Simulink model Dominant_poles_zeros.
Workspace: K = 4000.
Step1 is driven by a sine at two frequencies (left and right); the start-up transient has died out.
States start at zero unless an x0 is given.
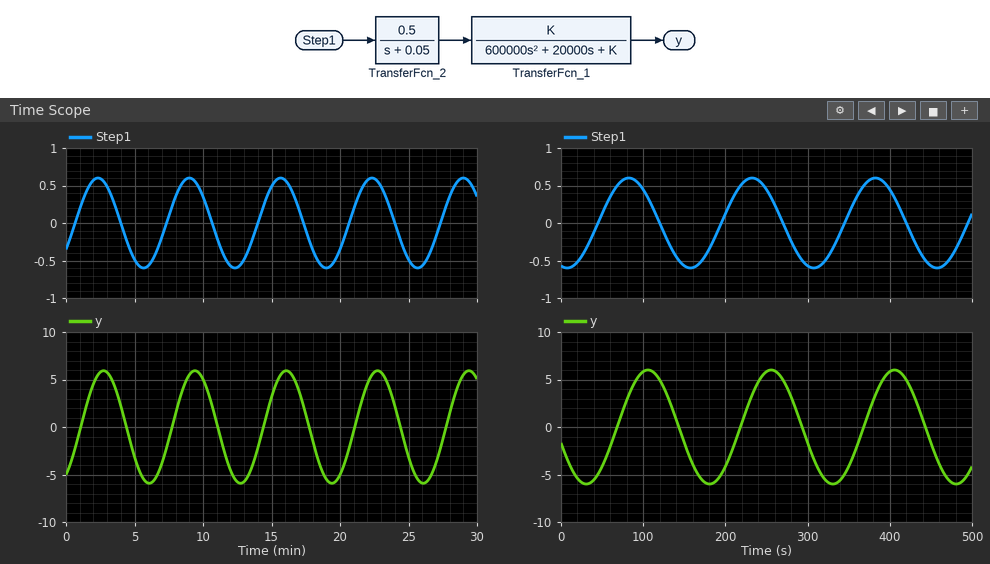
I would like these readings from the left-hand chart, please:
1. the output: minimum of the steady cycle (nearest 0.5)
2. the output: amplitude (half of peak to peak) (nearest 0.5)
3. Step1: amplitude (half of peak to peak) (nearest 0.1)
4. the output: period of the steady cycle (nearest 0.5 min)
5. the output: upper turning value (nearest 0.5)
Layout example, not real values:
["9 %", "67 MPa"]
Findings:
["-6.0", "6.0", "0.6", "6.5 min", "6.0"]
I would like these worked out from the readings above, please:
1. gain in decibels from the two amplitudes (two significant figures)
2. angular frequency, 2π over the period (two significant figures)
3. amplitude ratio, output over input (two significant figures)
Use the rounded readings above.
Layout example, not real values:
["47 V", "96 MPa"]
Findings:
["20 dB", "0.97 rad/min", "10.0"]
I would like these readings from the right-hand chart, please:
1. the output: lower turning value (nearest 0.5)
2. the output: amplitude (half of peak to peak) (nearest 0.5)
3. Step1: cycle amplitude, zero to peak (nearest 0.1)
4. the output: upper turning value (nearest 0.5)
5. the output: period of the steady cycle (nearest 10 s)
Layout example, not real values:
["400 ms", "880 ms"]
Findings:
["-6.0", "6.0", "0.6", "6.0", "150 s"]
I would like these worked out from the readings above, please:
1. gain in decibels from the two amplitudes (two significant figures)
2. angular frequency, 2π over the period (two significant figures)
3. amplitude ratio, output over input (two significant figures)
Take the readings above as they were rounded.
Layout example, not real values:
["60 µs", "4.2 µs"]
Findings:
["20 dB", "0.042 rad/s", "10.0"]
